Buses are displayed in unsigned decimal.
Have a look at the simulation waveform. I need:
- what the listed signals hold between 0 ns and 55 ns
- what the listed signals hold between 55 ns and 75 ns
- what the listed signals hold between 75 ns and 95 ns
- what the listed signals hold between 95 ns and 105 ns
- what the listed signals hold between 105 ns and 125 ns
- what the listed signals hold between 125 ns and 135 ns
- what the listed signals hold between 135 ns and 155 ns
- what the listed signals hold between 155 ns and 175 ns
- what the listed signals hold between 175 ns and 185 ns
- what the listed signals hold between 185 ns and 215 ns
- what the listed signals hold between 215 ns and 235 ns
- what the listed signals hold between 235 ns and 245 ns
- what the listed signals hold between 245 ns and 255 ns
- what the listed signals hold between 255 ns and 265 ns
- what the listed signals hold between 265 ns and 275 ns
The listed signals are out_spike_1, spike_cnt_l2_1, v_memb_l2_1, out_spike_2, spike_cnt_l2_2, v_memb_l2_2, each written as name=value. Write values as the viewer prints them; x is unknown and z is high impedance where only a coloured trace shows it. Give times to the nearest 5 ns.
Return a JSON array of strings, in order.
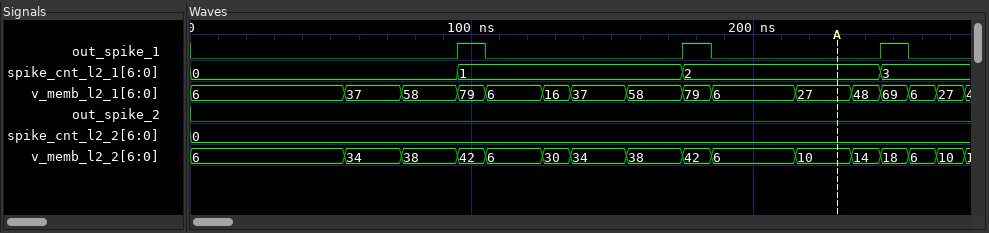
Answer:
["out_spike_1=0, spike_cnt_l2_1=0, v_memb_l2_1=6, out_spike_2=0, spike_cnt_l2_2=0, v_memb_l2_2=6", "out_spike_1=0, spike_cnt_l2_1=0, v_memb_l2_1=37, out_spike_2=0, spike_cnt_l2_2=0, v_memb_l2_2=34", "out_spike_1=0, spike_cnt_l2_1=0, v_memb_l2_1=58, out_spike_2=0, spike_cnt_l2_2=0, v_memb_l2_2=38", "out_spike_1=1, spike_cnt_l2_1=1, v_memb_l2_1=79, out_spike_2=0, spike_cnt_l2_2=0, v_memb_l2_2=42", "out_spike_1=0, spike_cnt_l2_1=1, v_memb_l2_1=6, out_spike_2=0, spike_cnt_l2_2=0, v_memb_l2_2=6", "out_spike_1=0, spike_cnt_l2_1=1, v_memb_l2_1=16, out_spike_2=0, spike_cnt_l2_2=0, v_memb_l2_2=30", "out_spike_1=0, spike_cnt_l2_1=1, v_memb_l2_1=37, out_spike_2=0, spike_cnt_l2_2=0, v_memb_l2_2=34", "out_spike_1=0, spike_cnt_l2_1=1, v_memb_l2_1=58, out_spike_2=0, spike_cnt_l2_2=0, v_memb_l2_2=38", "out_spike_1=1, spike_cnt_l2_1=2, v_memb_l2_1=79, out_spike_2=0, spike_cnt_l2_2=0, v_memb_l2_2=42", "out_spike_1=0, spike_cnt_l2_1=2, v_memb_l2_1=6, out_spike_2=0, spike_cnt_l2_2=0, v_memb_l2_2=6", "out_spike_1=0, spike_cnt_l2_1=2, v_memb_l2_1=27, out_spike_2=0, spike_cnt_l2_2=0, v_memb_l2_2=10", "out_spike_1=0, spike_cnt_l2_1=2, v_memb_l2_1=48, out_spike_2=0, spike_cnt_l2_2=0, v_memb_l2_2=14", "out_spike_1=1, spike_cnt_l2_1=3, v_memb_l2_1=69, out_spike_2=0, spike_cnt_l2_2=0, v_memb_l2_2=18", "out_spike_1=0, spike_cnt_l2_1=3, v_memb_l2_1=6, out_spike_2=0, spike_cnt_l2_2=0, v_memb_l2_2=6", "out_spike_1=0, spike_cnt_l2_1=3, v_memb_l2_1=27, out_spike_2=0, spike_cnt_l2_2=0, v_memb_l2_2=10"]
